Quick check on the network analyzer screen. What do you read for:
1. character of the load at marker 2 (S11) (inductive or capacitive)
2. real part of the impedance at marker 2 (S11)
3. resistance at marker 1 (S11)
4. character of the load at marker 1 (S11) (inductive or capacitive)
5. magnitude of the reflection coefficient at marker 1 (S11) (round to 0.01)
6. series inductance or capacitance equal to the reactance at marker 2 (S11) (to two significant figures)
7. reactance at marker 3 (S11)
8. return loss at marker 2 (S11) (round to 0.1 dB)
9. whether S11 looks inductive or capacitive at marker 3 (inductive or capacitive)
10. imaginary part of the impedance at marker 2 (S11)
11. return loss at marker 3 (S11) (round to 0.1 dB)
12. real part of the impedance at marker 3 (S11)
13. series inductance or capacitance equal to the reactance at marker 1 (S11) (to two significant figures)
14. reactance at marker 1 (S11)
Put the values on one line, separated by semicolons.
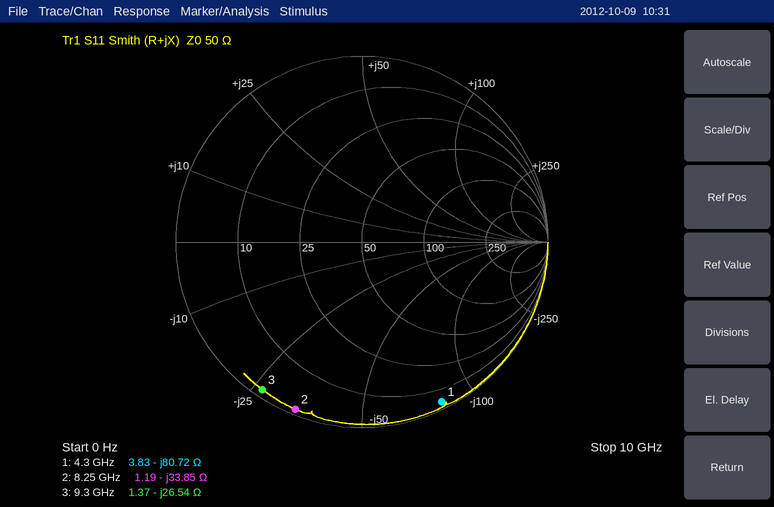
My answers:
capacitive; 1.19 Ω; 3.83 Ω; capacitive; 0.96; 570 fF; -26.54 Ω; 0.3 dB; capacitive; -33.85 Ω; 0.4 dB; 1.37 Ω; 460 fF; -80.72 Ω
